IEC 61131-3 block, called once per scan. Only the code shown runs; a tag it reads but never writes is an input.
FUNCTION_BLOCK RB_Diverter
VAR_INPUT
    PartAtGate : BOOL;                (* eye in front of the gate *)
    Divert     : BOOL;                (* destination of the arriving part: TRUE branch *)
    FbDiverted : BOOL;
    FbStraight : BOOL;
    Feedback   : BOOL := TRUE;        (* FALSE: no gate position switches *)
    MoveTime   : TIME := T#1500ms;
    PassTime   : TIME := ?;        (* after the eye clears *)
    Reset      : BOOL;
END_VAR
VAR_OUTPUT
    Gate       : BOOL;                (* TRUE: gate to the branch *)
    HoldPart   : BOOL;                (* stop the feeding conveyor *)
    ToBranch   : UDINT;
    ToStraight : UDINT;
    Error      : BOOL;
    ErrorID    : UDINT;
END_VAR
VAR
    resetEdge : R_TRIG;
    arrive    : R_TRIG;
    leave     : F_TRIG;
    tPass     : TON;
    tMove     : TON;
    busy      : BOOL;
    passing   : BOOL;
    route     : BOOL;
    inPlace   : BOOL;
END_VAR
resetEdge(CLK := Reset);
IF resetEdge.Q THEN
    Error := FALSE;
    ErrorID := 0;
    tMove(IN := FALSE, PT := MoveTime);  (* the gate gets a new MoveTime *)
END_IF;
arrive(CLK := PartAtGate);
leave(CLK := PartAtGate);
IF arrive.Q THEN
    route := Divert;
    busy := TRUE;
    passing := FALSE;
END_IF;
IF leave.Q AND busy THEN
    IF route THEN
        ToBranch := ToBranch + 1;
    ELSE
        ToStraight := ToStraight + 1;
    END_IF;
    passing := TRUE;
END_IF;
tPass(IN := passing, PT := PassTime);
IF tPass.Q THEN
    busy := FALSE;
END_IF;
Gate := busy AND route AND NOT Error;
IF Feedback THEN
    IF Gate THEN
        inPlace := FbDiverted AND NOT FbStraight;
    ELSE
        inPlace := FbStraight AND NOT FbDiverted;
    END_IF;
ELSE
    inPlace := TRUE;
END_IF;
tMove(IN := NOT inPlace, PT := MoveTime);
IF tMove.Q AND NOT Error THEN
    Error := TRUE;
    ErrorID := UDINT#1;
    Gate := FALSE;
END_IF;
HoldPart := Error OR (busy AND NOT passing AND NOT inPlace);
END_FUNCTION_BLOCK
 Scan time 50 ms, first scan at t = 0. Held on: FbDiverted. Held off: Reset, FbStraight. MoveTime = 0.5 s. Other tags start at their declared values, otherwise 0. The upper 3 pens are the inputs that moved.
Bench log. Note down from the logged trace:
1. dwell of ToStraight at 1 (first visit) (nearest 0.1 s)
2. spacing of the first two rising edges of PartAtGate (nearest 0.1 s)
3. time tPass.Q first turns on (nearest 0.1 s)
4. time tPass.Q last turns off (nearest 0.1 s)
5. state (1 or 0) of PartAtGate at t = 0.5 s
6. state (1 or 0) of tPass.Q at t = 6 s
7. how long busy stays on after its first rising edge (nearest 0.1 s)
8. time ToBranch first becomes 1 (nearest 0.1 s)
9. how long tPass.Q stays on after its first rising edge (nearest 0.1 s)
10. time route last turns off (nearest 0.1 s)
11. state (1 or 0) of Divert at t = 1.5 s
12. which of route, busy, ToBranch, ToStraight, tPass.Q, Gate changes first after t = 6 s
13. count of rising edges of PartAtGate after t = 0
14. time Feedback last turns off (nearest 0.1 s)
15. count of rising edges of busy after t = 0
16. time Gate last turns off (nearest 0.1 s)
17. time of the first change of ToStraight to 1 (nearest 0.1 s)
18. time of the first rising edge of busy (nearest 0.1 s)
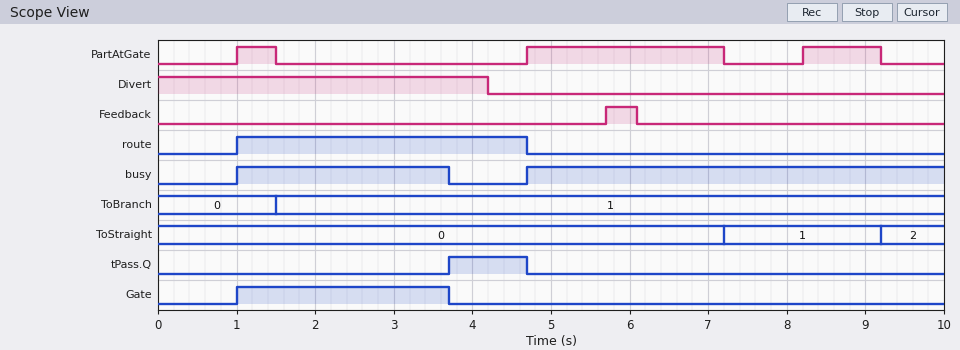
2.0 s
3.7 s
3.7 s
4.7 s
0
0
2.7 s
1.5 s
1.0 s
4.7 s
1
ToStraight
3
6.1 s
2
3.7 s
7.2 s
1.0 s
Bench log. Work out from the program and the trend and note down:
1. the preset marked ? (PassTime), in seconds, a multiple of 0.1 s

2.2 s
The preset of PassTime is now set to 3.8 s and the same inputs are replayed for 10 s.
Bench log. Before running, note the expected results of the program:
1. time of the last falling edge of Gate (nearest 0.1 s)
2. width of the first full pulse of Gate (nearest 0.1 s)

4.7 s
3.7 s
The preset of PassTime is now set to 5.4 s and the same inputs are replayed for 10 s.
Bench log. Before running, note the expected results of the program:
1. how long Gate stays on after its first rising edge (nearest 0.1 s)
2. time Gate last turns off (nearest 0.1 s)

3.7 s
4.7 s
